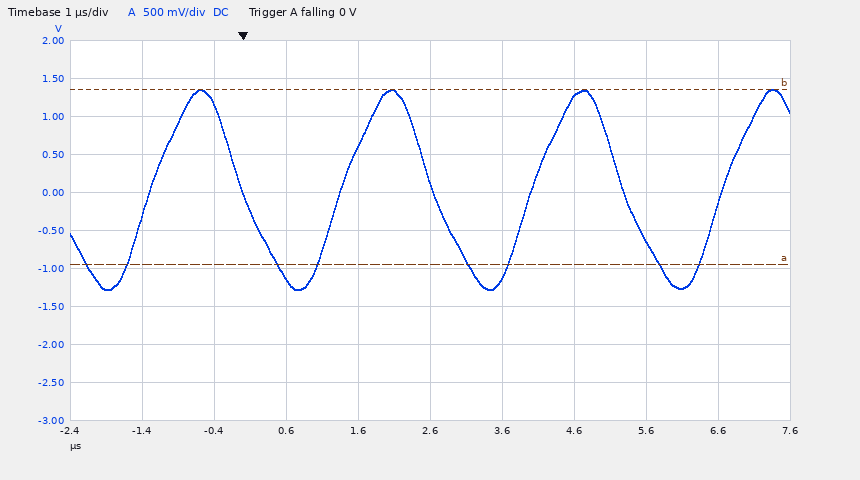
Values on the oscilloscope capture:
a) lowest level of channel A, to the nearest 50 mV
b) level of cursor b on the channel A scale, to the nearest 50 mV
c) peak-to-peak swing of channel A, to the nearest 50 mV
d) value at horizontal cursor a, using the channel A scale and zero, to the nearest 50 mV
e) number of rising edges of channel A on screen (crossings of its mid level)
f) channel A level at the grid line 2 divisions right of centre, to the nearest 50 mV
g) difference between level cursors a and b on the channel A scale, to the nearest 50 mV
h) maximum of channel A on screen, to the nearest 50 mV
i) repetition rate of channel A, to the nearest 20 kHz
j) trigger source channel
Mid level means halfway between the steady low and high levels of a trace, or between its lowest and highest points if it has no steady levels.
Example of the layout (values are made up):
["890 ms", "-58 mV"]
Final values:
["-1.30 V", "1.35 V", "2.65 V", "-950 mV", "4", "1.25 V", "2.30 V", "1.35 V", "380 kHz", "channel A"]
